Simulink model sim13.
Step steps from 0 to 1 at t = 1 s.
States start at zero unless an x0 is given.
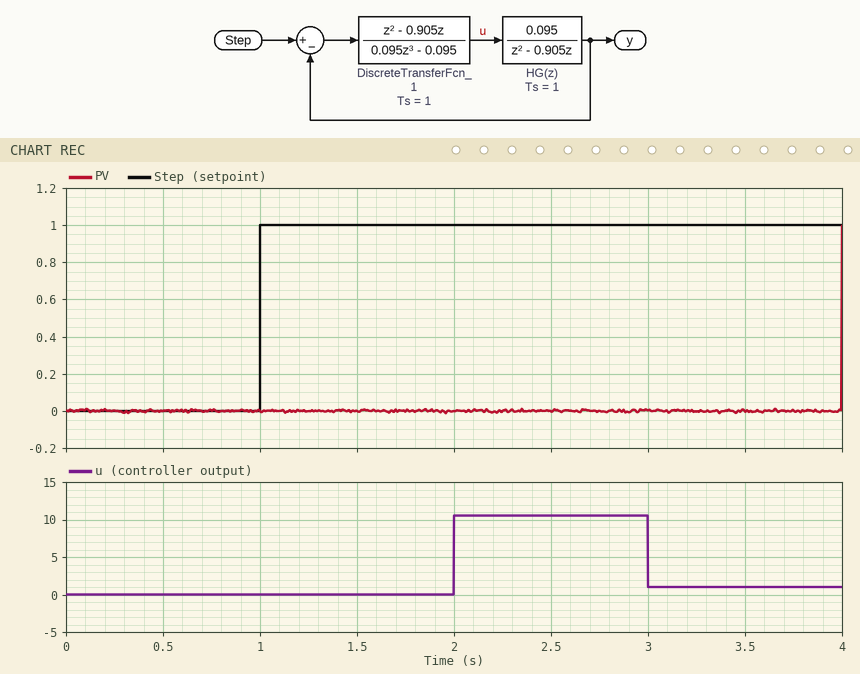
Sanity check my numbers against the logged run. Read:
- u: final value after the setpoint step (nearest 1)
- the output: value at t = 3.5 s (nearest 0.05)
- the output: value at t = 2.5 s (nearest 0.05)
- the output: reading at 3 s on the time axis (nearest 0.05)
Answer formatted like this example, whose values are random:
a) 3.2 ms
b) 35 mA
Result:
a) 1
b) 0.00
c) 0.00
d) 0.00
